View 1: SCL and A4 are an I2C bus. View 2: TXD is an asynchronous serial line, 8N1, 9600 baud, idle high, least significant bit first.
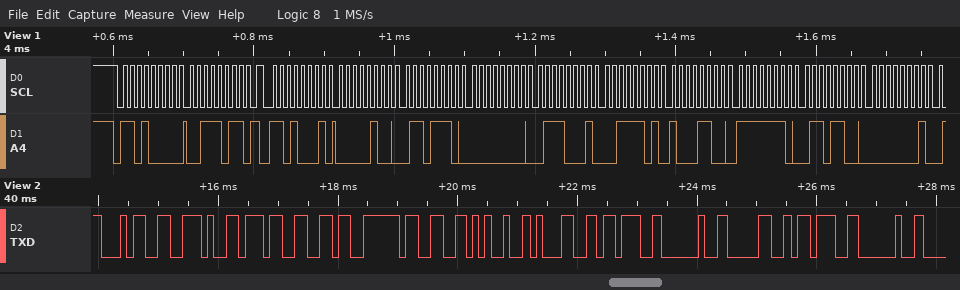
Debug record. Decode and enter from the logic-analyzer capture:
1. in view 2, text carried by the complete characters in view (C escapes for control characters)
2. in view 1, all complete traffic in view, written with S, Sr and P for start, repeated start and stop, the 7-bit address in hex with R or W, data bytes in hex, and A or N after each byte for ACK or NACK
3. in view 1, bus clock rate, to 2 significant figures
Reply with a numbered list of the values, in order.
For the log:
1. "4.763%1; 0; "
2. S 68W A 3B A Sr 68R A 04 A 6E A 00 A 71 A 3D A 8C A FE A 6C A 01 A
3. 100 kHz
